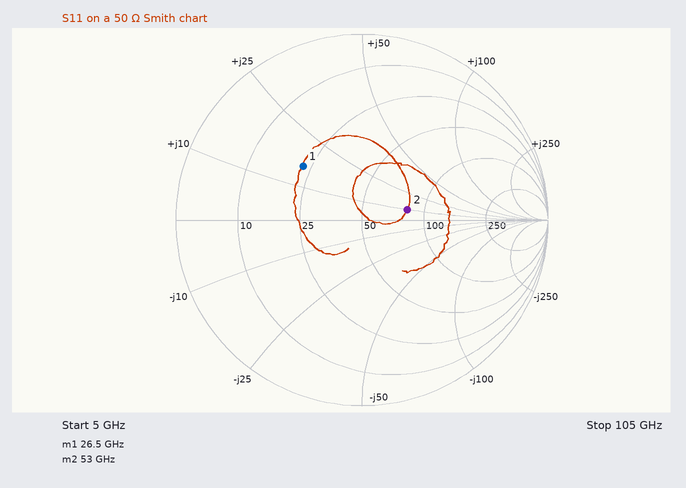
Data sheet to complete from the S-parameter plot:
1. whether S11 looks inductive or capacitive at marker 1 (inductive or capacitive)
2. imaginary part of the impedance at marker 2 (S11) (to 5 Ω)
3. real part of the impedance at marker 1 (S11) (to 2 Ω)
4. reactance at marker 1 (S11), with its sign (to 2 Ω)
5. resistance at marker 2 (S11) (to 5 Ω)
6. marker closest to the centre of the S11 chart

inductive
+10 Ω
22 Ω
+16 Ω
80 Ω
marker 2
